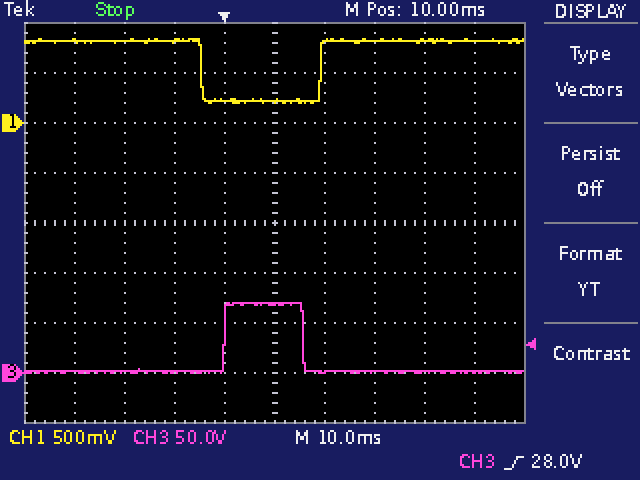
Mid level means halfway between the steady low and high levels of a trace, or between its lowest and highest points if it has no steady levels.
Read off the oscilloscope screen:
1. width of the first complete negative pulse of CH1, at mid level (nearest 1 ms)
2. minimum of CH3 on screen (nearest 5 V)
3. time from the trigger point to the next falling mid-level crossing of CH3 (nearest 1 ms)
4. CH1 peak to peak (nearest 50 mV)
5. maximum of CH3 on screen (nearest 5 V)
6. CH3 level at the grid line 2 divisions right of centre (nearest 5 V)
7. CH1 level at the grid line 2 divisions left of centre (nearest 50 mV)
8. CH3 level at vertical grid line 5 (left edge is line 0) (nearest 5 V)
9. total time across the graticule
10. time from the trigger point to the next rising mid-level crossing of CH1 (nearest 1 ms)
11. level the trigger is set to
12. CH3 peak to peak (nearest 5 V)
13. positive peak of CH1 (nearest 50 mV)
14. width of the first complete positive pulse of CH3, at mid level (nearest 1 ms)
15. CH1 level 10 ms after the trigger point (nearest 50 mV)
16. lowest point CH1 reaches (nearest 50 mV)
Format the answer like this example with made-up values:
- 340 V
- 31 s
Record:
- 24 ms
- 0 V
- 16 ms
- 650 mV
- 70 V
- 0 V
- 800 mV
- 70 V
- 100 ms
- 19 ms
- 28.0 V
- 70 V
- 850 mV
- 16 ms
- 200 mV
- 200 mV
